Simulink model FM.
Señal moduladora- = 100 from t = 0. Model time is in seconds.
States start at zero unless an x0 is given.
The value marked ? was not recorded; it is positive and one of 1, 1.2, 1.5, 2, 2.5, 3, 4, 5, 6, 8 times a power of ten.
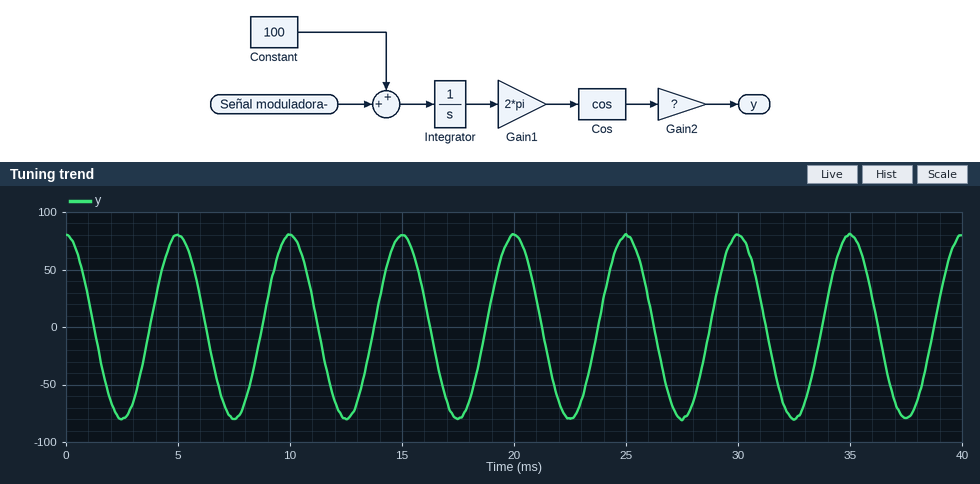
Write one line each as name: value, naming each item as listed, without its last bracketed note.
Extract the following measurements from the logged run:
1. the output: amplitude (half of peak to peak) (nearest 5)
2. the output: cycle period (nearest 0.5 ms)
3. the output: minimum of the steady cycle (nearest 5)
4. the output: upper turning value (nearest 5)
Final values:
the output: amplitude (half of peak to peak): 80
the output: cycle period: 5.0 ms
the output: minimum of the steady cycle: -80
the output: upper turning value: 80
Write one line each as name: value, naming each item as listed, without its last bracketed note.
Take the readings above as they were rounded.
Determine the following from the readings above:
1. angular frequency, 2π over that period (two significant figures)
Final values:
angular frequency, 2π over that period: 1.3 rad/ms
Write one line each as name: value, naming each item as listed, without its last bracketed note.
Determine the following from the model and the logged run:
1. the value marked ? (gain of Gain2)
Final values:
the value marked ?: 80
